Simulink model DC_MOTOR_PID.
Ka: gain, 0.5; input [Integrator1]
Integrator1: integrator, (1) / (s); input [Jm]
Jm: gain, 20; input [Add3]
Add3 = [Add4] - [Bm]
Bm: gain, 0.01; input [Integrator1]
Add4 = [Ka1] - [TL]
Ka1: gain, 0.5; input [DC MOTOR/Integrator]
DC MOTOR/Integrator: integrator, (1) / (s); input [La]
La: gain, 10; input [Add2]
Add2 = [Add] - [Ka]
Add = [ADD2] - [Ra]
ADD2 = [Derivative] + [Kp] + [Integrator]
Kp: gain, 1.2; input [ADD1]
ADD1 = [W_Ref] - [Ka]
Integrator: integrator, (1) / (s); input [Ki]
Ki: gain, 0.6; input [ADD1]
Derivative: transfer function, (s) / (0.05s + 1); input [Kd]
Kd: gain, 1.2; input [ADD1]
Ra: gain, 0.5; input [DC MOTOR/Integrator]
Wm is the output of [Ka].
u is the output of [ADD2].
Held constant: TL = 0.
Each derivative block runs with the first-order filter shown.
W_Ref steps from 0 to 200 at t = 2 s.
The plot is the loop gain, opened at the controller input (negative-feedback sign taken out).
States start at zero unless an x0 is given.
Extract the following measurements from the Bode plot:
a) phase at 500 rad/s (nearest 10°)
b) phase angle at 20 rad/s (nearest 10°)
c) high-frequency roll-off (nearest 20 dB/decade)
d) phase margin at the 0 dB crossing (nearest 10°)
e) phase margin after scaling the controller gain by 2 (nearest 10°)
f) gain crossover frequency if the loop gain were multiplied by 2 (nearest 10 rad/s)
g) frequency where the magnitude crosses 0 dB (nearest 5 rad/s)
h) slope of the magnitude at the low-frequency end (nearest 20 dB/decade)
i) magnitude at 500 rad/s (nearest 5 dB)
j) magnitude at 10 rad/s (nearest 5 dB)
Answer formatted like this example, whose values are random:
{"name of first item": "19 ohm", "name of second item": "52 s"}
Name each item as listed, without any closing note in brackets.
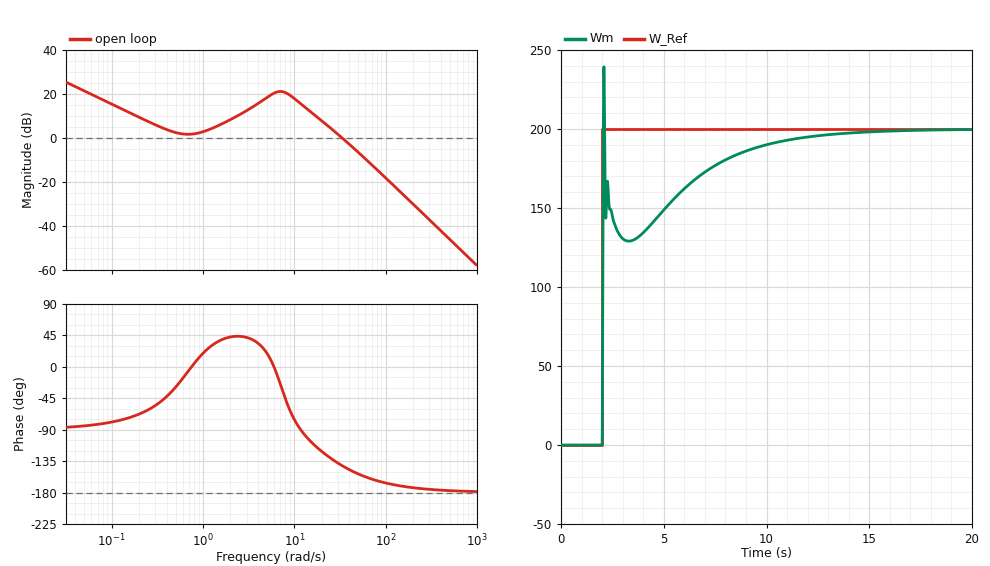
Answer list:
{"phase at 500 rad/s": "-180°", "phase angle at 20 rad/s": "-120°", "high-frequency roll-off": "-40 dB/decade", "phase margin at the 0 dB crossing": "40°", "phase margin after scaling the controller gain by 2": "30°", "gain crossover frequency if the loop gain were multiplied by 2": "50 rad/s", "frequency where the magnitude crosses 0 dB": "35 rad/s", "slope of the magnitude at the low-frequency end": "-20 dB/decade", "magnitude at 500 rad/s": "-45 dB", "magnitude at 10 rad/s": "20 dB"}
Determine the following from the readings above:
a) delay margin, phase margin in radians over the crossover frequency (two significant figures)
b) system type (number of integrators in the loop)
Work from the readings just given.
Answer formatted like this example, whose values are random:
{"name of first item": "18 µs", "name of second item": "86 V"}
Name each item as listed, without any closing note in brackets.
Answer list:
{"delay margin, phase margin in radians over the crossover frequency": "0.020 s", "system type": "1"}
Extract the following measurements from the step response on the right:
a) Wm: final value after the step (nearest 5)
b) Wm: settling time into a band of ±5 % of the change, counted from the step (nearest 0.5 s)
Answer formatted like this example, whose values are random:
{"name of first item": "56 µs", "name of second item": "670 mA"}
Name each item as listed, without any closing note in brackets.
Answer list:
{"Wm: final value after the step": "200", "Wm: settling time into a band of ±5 % of the change, counted from the step": "8.0 s"}
